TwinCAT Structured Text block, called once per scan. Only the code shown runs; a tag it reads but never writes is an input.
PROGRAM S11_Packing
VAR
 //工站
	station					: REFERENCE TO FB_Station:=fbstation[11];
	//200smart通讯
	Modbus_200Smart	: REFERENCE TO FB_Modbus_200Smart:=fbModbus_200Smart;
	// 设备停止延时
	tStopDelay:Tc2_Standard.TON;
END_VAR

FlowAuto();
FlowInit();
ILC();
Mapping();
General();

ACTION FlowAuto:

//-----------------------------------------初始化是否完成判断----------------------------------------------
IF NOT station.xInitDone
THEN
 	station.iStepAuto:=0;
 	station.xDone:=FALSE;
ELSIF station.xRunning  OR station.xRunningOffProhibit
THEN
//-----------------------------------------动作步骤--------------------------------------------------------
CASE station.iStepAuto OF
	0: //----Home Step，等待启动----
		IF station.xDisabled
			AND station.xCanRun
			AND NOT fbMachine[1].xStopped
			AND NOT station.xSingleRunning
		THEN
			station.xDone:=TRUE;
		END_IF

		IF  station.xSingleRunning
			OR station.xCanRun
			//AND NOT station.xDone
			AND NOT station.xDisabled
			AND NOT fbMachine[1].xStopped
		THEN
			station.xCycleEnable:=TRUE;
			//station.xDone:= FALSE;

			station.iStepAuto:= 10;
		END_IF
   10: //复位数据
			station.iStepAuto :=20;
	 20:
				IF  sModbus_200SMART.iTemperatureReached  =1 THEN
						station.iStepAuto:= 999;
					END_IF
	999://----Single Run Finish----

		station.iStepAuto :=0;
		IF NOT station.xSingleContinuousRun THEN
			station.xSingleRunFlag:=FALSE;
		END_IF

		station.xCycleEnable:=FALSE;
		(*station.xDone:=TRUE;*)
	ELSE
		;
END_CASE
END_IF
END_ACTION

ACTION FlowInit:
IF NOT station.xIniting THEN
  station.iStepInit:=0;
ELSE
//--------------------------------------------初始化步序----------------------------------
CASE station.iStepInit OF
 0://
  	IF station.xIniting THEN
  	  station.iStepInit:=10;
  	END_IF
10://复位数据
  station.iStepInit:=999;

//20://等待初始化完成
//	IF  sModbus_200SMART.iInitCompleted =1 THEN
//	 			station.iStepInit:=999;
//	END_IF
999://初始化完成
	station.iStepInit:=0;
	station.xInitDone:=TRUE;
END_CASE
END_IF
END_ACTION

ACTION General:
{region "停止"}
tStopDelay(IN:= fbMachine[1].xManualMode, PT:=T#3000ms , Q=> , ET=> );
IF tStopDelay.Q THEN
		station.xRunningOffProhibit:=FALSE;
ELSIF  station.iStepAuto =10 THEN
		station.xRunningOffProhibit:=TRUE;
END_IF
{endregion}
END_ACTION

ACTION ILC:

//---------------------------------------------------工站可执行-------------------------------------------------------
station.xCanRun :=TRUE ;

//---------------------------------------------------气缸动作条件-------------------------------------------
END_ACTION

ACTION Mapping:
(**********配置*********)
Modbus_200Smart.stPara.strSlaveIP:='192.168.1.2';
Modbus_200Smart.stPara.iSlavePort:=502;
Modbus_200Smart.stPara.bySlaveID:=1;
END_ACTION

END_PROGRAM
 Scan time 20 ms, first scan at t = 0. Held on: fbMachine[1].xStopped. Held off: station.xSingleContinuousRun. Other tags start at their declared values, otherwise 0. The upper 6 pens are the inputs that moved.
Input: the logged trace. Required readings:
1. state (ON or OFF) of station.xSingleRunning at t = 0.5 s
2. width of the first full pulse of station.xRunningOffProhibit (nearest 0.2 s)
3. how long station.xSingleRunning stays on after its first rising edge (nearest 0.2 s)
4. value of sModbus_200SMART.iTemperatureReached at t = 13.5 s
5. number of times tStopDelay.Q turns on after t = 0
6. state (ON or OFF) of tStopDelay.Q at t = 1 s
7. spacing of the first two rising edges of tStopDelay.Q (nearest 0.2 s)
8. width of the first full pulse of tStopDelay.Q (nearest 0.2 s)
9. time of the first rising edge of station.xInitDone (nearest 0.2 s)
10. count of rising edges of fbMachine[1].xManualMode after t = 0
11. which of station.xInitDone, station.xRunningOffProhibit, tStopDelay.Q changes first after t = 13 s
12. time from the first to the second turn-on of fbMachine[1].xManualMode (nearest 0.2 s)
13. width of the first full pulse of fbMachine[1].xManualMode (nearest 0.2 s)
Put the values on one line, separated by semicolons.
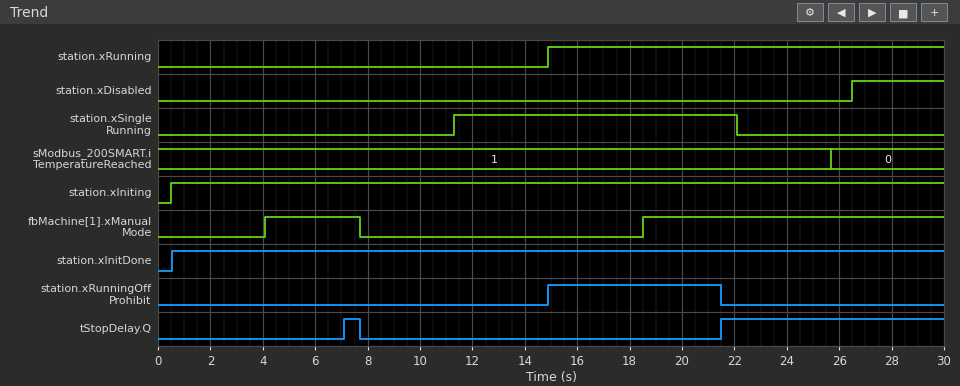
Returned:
OFF; 6.6 s; 10.8 s; 1; 2; OFF; 14.4 s; 0.6 s; 0.6 s; 2; station.xRunningOffProhibit; 14.4 s; 3.6 s
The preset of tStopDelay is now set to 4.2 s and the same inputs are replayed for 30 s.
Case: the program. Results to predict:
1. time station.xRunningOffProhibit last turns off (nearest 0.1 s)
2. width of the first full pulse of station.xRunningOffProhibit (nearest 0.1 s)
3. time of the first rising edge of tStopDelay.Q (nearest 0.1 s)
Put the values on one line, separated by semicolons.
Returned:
22.7 s; 7.8 s; 22.7 s
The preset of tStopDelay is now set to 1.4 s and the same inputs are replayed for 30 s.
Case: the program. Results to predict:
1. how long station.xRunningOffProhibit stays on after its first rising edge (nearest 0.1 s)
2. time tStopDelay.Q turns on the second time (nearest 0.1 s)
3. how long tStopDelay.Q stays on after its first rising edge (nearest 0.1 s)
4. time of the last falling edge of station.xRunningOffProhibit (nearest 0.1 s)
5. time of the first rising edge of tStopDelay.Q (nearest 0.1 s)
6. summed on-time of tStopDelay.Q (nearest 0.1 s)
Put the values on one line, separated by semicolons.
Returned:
5.0 s; 19.9 s; 2.2 s; 19.9 s; 5.5 s; 12.3 s
